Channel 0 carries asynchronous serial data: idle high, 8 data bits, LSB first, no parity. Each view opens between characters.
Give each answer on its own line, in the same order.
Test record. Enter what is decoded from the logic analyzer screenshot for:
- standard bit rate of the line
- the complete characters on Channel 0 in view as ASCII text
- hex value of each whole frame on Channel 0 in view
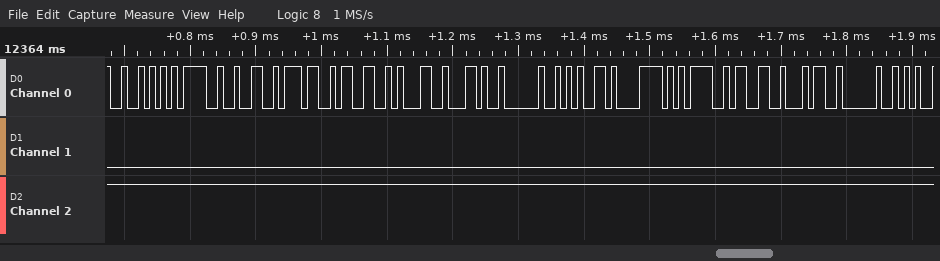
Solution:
115200 baud
"R=2731, ex=34 "
52, 3D, 32, 37, 33, 31, 2C, 20, 65, 78, 3D, 33, 34, 20
